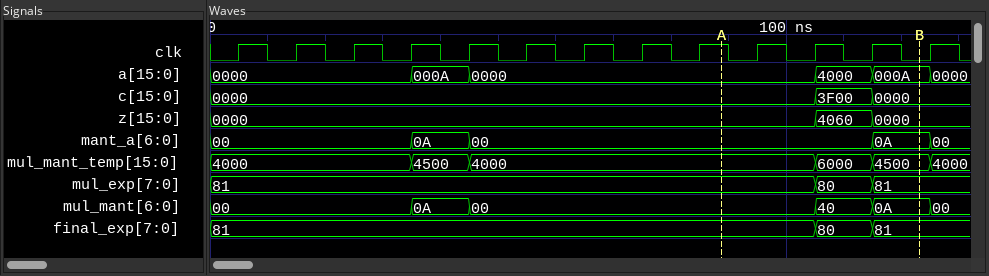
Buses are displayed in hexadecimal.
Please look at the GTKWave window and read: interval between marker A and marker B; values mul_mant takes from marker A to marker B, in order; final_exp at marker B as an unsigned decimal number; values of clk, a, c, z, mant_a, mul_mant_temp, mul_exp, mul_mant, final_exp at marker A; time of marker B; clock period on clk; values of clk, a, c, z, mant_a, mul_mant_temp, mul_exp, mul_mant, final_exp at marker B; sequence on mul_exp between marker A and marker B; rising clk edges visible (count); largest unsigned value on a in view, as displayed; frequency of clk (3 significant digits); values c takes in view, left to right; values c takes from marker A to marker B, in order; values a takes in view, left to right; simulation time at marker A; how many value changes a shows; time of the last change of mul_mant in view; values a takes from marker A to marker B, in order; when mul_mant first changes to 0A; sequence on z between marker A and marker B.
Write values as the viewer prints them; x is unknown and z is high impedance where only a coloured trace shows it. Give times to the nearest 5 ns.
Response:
35 ns
00, 40, 0A
129
clk=1, a=0000, c=0000, z=0000, mant_a=00, mul_mant_temp=4000, mul_exp=81, mul_mant=00, final_exp=81
125 ns
10 ns
clk=0, a=000A, c=0000, z=0000, mant_a=0A, mul_mant_temp=4500, mul_exp=81, mul_mant=0A, final_exp=81
81, 80, 81
13
4000
100 MHz
0000, 3F00, 0000
0000, 3F00, 0000
0000, 000A, 0000, 4000, 000A, 0000
90 ns
5
125 ns
0000, 4000, 000A
35 ns
0000, 4060, 0000
